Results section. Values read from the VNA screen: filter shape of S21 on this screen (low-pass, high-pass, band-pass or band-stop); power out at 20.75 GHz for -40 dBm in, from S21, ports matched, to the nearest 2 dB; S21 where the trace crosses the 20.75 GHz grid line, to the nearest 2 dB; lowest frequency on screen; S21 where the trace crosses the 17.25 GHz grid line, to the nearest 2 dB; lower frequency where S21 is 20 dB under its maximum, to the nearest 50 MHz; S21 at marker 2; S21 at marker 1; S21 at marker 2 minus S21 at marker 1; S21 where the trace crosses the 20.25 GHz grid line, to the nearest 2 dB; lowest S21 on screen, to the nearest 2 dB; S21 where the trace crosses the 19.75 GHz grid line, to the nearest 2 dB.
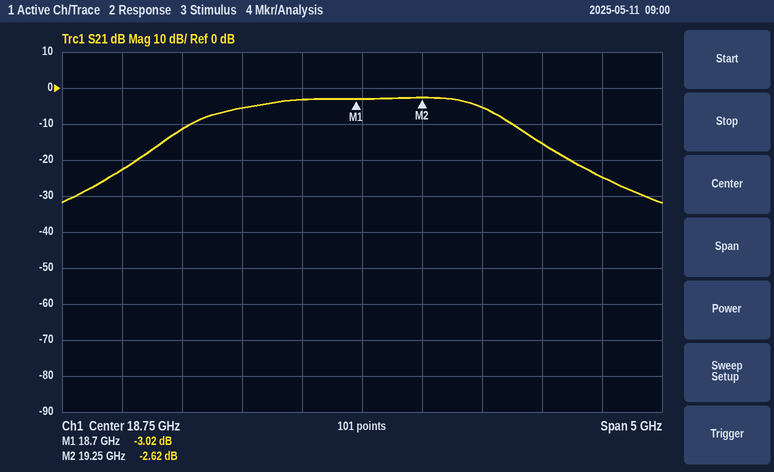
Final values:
band-pass
-64 dBm
-24 dB
16.25 GHz
-12 dB
16.75 GHz
-2.62 dB
-3.02 dB
0.40 dB
-16 dB
-32 dB
-6 dB
